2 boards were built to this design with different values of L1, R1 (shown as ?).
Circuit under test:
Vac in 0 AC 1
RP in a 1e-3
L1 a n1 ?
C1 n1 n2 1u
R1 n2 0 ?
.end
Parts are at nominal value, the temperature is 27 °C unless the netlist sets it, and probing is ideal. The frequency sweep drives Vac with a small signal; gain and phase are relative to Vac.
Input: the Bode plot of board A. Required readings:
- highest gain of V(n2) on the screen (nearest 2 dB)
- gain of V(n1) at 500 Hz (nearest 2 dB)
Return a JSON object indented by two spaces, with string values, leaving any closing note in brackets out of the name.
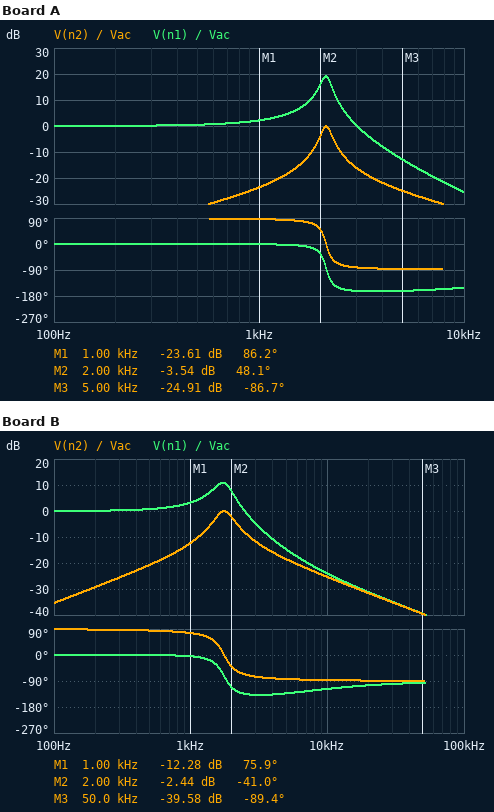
{
  "highest gain of V(n2) on the screen": "0 dB",
  "gain of V(n1) at 500 Hz": "0 dB"
}
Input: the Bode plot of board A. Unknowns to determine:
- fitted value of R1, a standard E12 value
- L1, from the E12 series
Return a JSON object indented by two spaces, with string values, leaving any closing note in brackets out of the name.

{
  "fitted value of R1, a standard E12 value": "8.2 Ω",
  "L1, from the E12 series": "5.6 mH"
}
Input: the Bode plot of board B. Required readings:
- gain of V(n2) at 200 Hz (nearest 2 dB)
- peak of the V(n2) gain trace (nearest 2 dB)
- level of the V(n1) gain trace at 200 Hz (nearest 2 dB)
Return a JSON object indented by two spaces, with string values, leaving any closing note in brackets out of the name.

{
  "gain of V(n2) at 200 Hz": "-30 dB",
  "peak of the V(n2) gain trace": "0 dB",
  "level of the V(n1) gain trace at 200 Hz": "0 dB"
}
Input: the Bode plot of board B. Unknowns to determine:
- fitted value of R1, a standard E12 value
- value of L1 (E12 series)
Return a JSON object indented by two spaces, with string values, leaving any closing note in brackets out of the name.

{
  "fitted value of R1, a standard E12 value": "27 Ω",
  "value of L1": "8.2 mH"
}
